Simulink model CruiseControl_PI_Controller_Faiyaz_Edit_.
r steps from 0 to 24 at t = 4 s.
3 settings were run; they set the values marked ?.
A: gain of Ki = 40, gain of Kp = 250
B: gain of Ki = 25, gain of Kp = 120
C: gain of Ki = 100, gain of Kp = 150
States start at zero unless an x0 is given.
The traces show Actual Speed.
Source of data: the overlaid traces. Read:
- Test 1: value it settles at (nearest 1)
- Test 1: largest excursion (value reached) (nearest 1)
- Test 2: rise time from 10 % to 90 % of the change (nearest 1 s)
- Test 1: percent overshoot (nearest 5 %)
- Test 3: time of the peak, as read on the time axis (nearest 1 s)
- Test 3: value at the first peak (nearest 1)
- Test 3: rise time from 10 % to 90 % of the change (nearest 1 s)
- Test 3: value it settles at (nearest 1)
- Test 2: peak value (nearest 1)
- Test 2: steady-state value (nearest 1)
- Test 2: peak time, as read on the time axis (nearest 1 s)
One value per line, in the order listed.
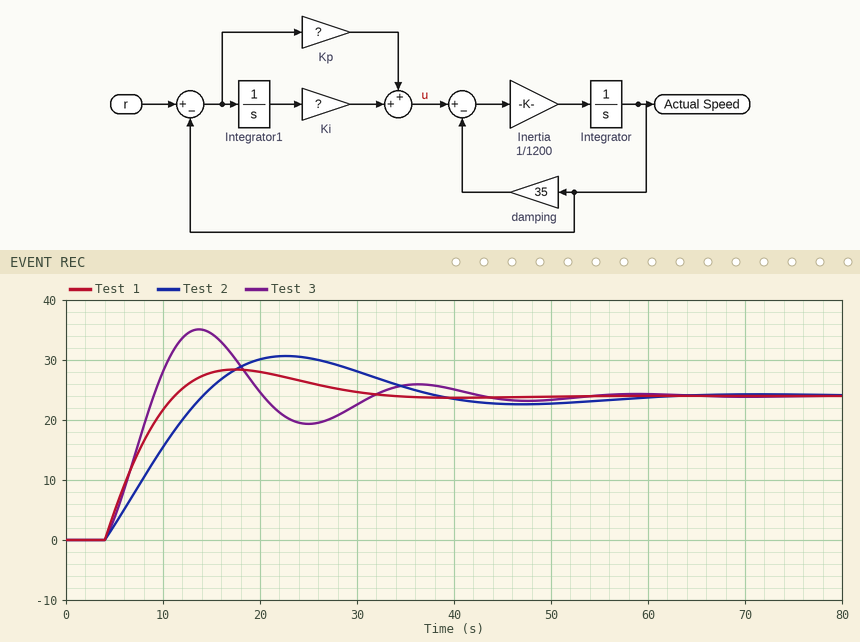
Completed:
24
28
8 s
20 %
14 s
35
4 s
24
31
24
23 s
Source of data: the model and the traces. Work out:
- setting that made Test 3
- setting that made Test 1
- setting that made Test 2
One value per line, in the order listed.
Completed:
C
A
B
